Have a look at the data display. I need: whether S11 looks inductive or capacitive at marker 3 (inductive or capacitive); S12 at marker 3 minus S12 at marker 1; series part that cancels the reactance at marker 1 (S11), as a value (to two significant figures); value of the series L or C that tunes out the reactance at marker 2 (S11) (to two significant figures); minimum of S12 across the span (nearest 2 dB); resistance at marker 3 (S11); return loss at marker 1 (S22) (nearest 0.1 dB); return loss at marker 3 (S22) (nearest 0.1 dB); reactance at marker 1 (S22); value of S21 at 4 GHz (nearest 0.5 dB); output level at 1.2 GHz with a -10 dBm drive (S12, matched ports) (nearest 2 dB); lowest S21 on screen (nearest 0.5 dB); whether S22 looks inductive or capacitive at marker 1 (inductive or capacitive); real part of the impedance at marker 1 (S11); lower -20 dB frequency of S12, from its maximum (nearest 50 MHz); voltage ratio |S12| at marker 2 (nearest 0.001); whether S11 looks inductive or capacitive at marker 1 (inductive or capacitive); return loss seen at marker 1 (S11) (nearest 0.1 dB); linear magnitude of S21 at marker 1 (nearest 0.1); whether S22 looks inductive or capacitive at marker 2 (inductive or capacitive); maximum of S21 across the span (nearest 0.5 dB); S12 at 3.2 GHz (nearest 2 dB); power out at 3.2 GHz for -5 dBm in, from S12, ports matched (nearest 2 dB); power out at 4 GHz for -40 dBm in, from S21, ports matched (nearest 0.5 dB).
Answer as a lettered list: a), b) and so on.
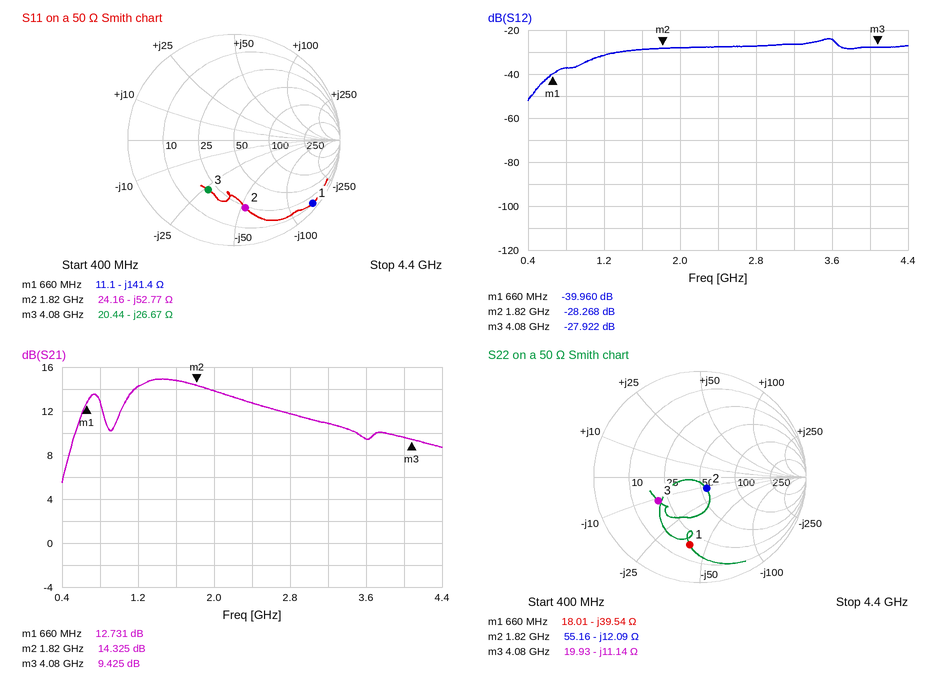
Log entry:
a) capacitive
b) 12.038 dB
c) 34 nH
d) 4.6 nH
e) -52 dB
f) 20.44 Ω
g) 3.8 dB
h) 6.9 dB
i) -39.54 Ω
j) 9.5 dB
k) -42 dBm
l) 5.5 dB
m) capacitive
n) 11.1 Ω
o) 550 MHz
p) 0.039
q) capacitive
r) 0.4 dB
s) 4.3
t) capacitive
u) 15.0 dB
v) -26 dB
w) -32 dBm
x) -30.5 dBm
